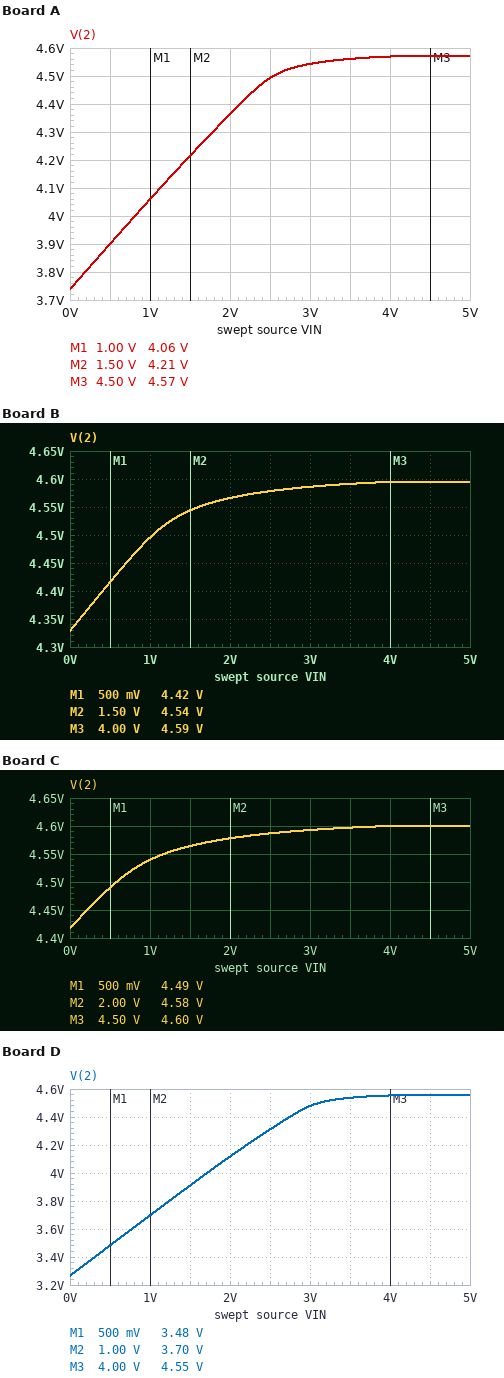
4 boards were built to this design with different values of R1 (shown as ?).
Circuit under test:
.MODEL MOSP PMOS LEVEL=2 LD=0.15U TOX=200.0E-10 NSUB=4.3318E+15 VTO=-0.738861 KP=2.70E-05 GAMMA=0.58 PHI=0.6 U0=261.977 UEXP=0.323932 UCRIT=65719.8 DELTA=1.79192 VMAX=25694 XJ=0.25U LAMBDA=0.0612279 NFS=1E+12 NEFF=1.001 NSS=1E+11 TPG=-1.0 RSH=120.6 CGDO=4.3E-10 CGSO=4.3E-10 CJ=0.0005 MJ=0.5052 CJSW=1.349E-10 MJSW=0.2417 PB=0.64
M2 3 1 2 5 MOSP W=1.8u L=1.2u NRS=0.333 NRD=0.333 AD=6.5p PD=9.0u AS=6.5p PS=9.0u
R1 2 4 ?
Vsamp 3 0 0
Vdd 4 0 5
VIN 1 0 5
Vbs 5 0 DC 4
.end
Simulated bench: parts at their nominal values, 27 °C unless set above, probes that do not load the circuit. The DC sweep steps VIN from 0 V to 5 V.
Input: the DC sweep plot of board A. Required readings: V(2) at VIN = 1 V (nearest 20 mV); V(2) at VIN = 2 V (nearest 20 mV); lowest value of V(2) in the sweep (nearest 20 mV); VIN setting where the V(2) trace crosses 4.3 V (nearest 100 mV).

4.06 V
4.36 V
3.74 V
1.8 V
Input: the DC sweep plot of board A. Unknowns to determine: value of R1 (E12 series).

12 kΩ
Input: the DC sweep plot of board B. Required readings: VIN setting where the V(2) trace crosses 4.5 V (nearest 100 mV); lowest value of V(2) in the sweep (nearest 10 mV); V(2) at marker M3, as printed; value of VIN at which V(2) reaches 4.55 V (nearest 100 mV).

1.0 V
4.33 V
4.59 V
1.6 V
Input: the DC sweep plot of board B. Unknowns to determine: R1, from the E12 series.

4.7 kΩ
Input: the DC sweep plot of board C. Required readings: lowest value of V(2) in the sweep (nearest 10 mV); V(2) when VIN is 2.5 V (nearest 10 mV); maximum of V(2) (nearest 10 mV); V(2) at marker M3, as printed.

4.42 V
4.59 V
4.60 V
4.60 V
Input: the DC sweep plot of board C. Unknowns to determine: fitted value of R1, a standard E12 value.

3.9 kΩ
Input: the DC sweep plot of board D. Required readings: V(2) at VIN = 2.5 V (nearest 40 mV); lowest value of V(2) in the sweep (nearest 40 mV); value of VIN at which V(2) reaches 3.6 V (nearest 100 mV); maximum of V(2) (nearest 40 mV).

4.32 V
3.28 V
800 mV
4.56 V
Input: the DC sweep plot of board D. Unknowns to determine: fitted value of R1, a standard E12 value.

22 kΩ
